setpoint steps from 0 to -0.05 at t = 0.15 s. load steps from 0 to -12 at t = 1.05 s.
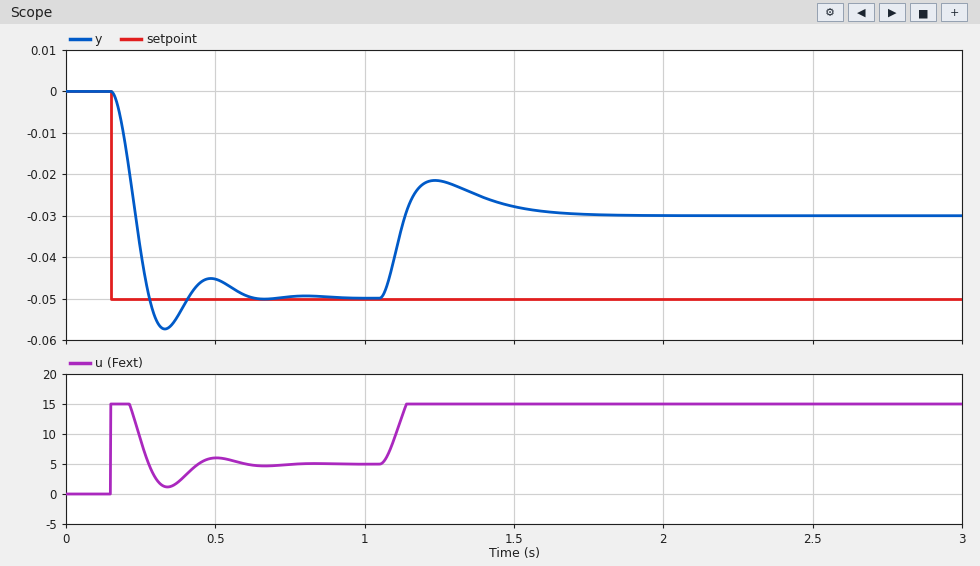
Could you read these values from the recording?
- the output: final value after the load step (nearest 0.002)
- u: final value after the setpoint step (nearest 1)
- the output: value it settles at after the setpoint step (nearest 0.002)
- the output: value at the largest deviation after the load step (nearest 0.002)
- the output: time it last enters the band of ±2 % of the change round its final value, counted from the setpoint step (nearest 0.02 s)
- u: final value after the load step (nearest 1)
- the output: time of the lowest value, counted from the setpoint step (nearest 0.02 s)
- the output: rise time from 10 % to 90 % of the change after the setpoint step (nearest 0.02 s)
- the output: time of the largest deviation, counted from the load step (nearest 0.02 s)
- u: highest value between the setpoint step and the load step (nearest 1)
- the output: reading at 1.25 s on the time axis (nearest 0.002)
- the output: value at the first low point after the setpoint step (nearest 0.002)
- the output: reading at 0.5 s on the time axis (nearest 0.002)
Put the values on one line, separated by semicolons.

-0.030; 5; -0.050; -0.022; 0.44 s; 15; 0.18 s; 0.08 s; 0.18 s; 15; -0.022; -0.058; -0.046
